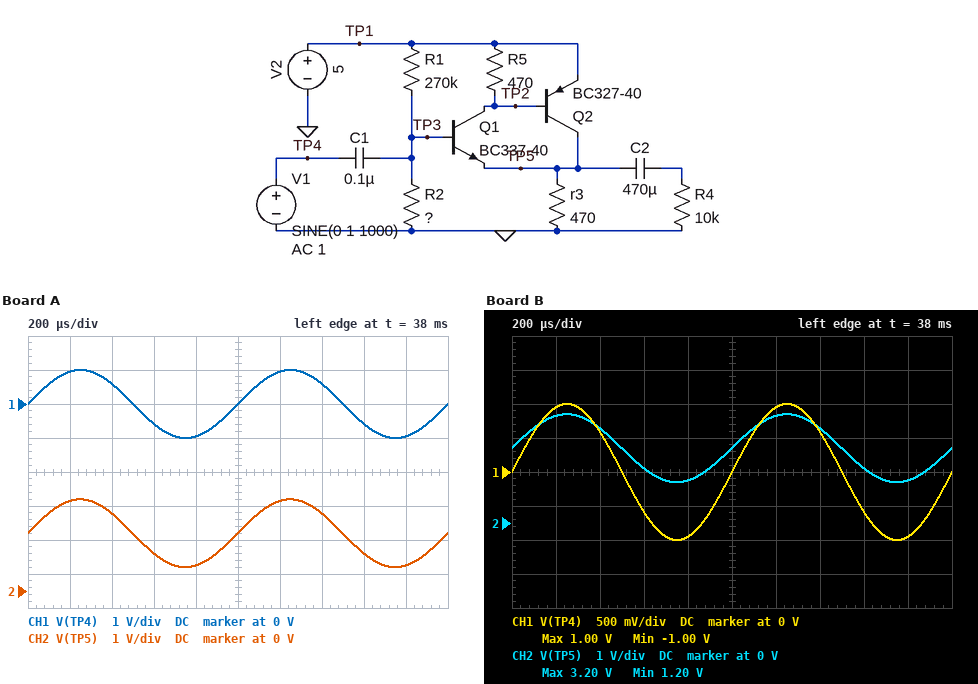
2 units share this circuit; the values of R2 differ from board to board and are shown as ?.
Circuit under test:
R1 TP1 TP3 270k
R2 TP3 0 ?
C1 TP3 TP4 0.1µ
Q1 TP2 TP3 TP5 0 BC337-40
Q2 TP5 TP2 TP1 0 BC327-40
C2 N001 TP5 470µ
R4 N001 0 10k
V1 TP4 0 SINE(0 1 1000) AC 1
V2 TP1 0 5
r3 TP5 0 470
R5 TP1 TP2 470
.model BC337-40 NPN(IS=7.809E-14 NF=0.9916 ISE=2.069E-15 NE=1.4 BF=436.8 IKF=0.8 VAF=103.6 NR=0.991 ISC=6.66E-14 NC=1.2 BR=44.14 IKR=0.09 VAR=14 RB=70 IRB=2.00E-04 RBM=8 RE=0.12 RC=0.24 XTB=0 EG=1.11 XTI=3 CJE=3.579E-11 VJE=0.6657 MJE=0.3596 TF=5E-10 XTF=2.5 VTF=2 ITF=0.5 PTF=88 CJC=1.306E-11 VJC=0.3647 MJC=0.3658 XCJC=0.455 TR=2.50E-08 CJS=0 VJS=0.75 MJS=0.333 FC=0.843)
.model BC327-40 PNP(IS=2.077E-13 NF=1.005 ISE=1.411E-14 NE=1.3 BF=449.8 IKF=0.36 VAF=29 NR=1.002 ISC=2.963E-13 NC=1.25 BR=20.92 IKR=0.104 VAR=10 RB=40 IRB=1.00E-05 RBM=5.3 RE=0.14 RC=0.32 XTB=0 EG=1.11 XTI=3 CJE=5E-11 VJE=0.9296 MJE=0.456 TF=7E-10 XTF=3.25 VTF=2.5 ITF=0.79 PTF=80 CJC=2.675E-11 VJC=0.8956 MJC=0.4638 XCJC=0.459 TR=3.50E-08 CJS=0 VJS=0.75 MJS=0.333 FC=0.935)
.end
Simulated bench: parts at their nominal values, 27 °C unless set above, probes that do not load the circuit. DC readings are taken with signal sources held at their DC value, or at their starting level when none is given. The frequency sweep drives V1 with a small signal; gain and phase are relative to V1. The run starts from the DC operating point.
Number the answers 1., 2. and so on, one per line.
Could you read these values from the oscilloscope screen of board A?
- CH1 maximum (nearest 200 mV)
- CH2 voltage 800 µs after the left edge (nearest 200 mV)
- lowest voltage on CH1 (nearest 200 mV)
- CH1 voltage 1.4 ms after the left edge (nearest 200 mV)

1. 1.0 V
2. 800 mV
3. -1.0 V
4. 600 mV
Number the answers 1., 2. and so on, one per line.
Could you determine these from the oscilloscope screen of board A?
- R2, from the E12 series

1. 330 kΩ
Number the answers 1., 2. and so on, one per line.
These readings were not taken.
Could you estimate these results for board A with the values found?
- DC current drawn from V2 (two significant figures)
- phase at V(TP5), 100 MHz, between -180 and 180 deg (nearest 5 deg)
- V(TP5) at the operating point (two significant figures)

1. 3.6 mA
2. 20 deg
3. 1.7 V
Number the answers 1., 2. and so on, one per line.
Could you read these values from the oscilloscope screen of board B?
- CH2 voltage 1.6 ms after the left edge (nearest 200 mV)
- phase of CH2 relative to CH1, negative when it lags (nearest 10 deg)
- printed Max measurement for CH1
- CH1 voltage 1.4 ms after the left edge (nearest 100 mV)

1. 1.6 V
2. 0 deg
3. 1.00 V
4. 600 mV
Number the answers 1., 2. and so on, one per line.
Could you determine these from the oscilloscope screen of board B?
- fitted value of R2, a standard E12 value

1. 560 kΩ
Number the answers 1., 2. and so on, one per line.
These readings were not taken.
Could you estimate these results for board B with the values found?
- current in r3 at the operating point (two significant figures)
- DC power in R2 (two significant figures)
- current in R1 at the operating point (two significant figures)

1. 4.7 mA
2. 14 µW
3. 8.1 µA
